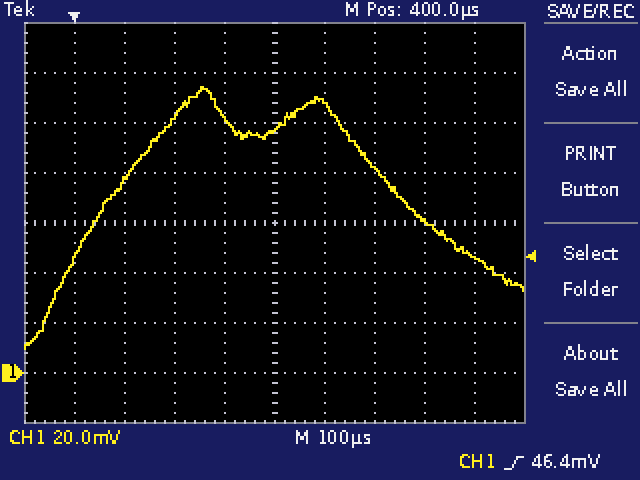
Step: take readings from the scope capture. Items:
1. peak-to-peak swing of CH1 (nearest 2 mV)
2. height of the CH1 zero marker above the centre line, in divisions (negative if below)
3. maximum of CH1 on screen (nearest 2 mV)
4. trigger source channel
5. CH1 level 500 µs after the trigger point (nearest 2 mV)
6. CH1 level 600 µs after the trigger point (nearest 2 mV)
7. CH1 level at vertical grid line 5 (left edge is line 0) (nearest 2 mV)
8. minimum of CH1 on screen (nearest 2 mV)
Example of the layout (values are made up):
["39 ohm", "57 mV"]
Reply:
["104 mV", "-3.0 div", "114 mV", "CH1", "108 mV", "82 mV", "98 mV", "10 mV"]
